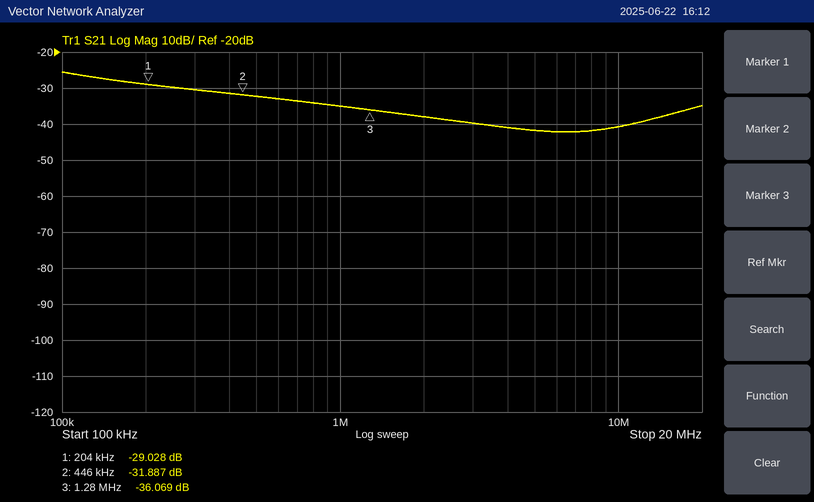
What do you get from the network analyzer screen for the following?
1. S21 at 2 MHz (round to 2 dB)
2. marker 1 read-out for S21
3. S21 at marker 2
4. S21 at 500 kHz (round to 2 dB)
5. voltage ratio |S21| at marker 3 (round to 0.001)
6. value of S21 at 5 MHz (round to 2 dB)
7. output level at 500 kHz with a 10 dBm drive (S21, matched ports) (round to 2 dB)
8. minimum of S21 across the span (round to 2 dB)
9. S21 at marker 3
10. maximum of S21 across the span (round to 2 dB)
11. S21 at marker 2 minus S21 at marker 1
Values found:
-38 dB
-29.028 dB
-31.887 dB
-32 dB
0.016
-42 dB
-22 dBm
-42 dB
-36.069 dB
-26 dB
-2.859 dB
